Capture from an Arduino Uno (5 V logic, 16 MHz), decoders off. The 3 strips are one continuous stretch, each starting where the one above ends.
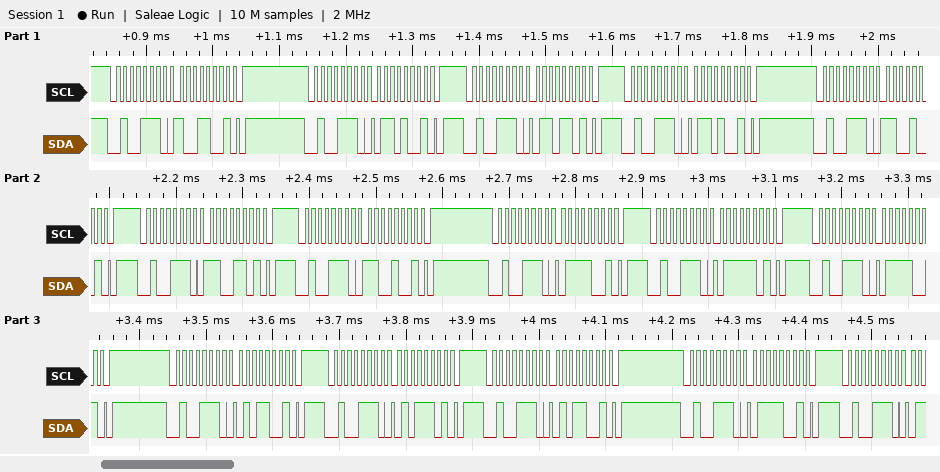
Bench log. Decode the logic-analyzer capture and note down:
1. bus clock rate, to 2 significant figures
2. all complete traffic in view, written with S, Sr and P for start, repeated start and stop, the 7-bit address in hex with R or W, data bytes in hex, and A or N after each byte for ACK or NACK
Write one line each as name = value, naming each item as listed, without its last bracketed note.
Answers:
bus clock rate, to 2 significant figures = 100 kHz
all complete traffic in view, written with S, Sr and P for start, repeated start and stop, the 7-bit address in hex with R or W, data bytes in hex, and A or N after each byte for ACK or NACK = S 27W A 99 A P S 27W A 69 A P S 27W A 6D A P S 27W A 69 A P S 27W A C9 A P S 27W A CD A P S 27W A C9 A P S 27W A 79 A P S 27W A 7D A P S 27W A 79 A P S 27W A 59 A P S 27W A 5D A P S 27W A 59 A P S 27W A 79 A P S 27W A
